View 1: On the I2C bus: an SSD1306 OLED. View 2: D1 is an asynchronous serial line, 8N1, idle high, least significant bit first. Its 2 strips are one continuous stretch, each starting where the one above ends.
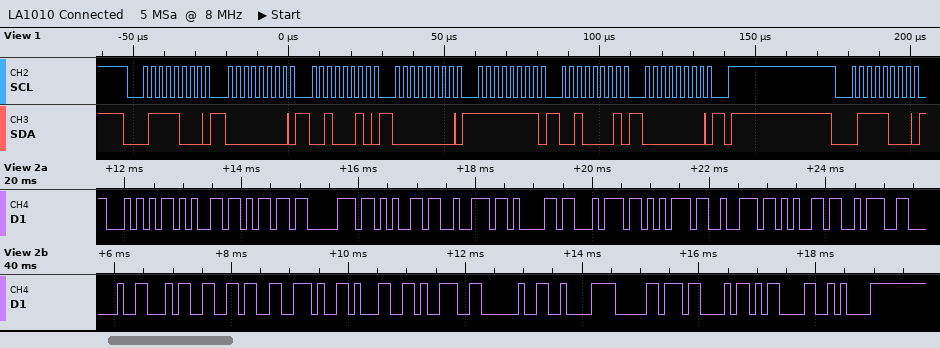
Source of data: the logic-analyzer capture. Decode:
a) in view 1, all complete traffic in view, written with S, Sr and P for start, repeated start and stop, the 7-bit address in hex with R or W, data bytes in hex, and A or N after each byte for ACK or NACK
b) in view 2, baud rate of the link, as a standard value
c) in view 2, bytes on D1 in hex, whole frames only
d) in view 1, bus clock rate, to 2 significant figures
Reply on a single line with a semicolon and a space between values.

S 3CW A 00 A 22 A 00 A FF A 21 A 00 A P S 3CW A; 9600 baud; 54 65 6D 70 65 72 61 74 75 72 65 3A 20 34 36 2E 31 39 20 C2 B0 43 0D 0A; 400 kHz
